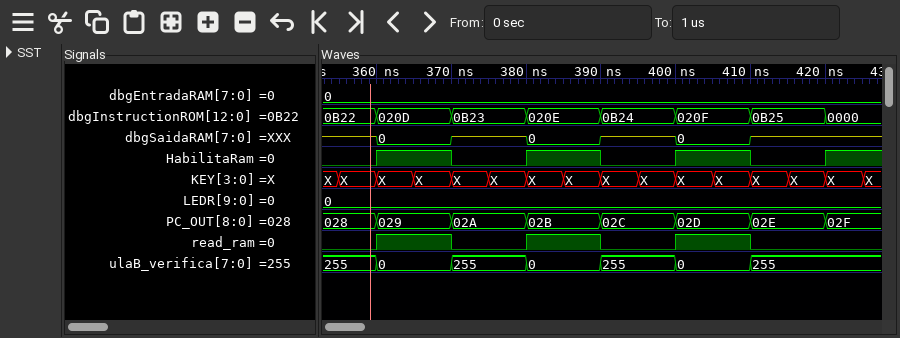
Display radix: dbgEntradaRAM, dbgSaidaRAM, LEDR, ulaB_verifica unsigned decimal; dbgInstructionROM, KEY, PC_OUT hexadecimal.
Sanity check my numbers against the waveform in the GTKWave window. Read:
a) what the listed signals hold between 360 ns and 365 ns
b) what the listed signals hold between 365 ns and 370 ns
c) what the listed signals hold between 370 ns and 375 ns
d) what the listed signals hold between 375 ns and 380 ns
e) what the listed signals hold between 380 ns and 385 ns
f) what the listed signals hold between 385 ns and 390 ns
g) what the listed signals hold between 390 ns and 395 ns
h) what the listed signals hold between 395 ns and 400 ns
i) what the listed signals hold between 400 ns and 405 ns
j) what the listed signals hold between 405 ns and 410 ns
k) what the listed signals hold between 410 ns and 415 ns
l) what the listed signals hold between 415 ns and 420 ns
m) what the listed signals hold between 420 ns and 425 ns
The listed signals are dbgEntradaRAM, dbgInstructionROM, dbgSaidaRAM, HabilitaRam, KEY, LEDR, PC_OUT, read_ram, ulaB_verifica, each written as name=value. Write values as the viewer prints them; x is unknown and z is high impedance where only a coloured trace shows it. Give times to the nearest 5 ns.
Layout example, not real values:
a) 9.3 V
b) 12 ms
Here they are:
a) dbgEntradaRAM=0, dbgInstructionROM=020D, dbgSaidaRAM=0, HabilitaRam=1, KEY=X, LEDR=0, PC_OUT=029, read_ram=1, ulaB_verifica=0
b) dbgEntradaRAM=0, dbgInstructionROM=020D, dbgSaidaRAM=0, HabilitaRam=1, KEY=X, LEDR=0, PC_OUT=029, read_ram=1, ulaB_verifica=0
c) dbgEntradaRAM=0, dbgInstructionROM=0B23, dbgSaidaRAM=z, HabilitaRam=0, KEY=X, LEDR=0, PC_OUT=02A, read_ram=0, ulaB_verifica=255
d) dbgEntradaRAM=0, dbgInstructionROM=0B23, dbgSaidaRAM=z, HabilitaRam=0, KEY=X, LEDR=0, PC_OUT=02A, read_ram=0, ulaB_verifica=255
e) dbgEntradaRAM=0, dbgInstructionROM=020E, dbgSaidaRAM=0, HabilitaRam=1, KEY=X, LEDR=0, PC_OUT=02B, read_ram=1, ulaB_verifica=0
f) dbgEntradaRAM=0, dbgInstructionROM=020E, dbgSaidaRAM=0, HabilitaRam=1, KEY=X, LEDR=0, PC_OUT=02B, read_ram=1, ulaB_verifica=0
g) dbgEntradaRAM=0, dbgInstructionROM=0B24, dbgSaidaRAM=z, HabilitaRam=0, KEY=X, LEDR=0, PC_OUT=02C, read_ram=0, ulaB_verifica=255
h) dbgEntradaRAM=0, dbgInstructionROM=0B24, dbgSaidaRAM=z, HabilitaRam=0, KEY=X, LEDR=0, PC_OUT=02C, read_ram=0, ulaB_verifica=255
i) dbgEntradaRAM=0, dbgInstructionROM=020F, dbgSaidaRAM=0, HabilitaRam=1, KEY=X, LEDR=0, PC_OUT=02D, read_ram=1, ulaB_verifica=0
j) dbgEntradaRAM=0, dbgInstructionROM=020F, dbgSaidaRAM=0, HabilitaRam=1, KEY=X, LEDR=0, PC_OUT=02D, read_ram=1, ulaB_verifica=0
k) dbgEntradaRAM=0, dbgInstructionROM=0B25, dbgSaidaRAM=z, HabilitaRam=0, KEY=X, LEDR=0, PC_OUT=02E, read_ram=0, ulaB_verifica=255
l) dbgEntradaRAM=0, dbgInstructionROM=0B25, dbgSaidaRAM=z, HabilitaRam=0, KEY=X, LEDR=0, PC_OUT=02E, read_ram=0, ulaB_verifica=255
m) dbgEntradaRAM=0, dbgInstructionROM=0000, dbgSaidaRAM=z, HabilitaRam=1, KEY=X, LEDR=0, PC_OUT=02F, read_ram=0, ulaB_verifica=255
